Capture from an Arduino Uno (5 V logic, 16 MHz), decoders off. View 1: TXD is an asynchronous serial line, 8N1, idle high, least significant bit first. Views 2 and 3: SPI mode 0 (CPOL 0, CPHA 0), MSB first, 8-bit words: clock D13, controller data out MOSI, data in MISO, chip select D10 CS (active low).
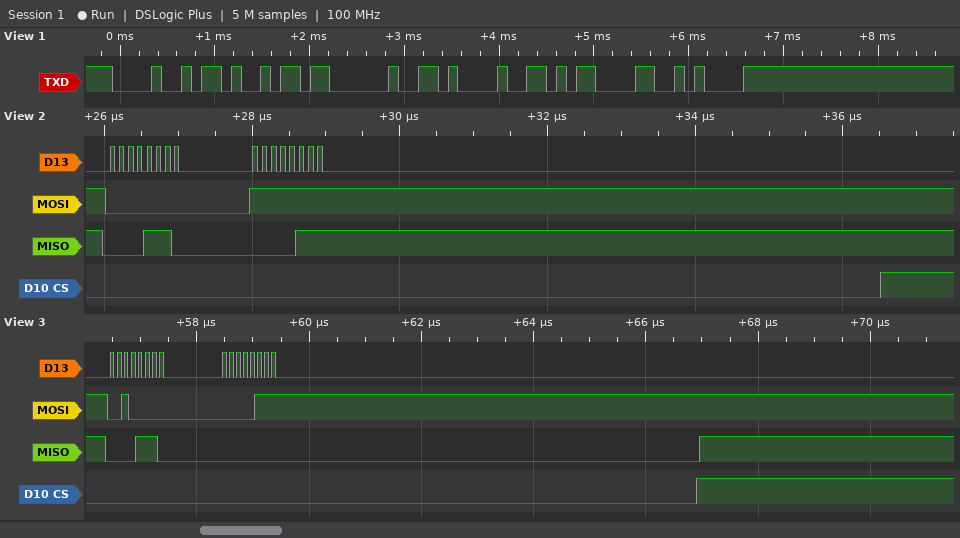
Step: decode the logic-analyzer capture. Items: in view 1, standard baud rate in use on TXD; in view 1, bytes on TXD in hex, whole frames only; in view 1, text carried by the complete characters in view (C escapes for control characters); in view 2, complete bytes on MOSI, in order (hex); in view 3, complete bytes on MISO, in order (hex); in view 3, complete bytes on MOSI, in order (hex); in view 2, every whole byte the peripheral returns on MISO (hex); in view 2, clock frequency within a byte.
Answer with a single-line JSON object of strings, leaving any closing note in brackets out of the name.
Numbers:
{"in view 1, standard baud rate in use on TXD": "9600 baud", "in view 1, bytes on TXD in hex, whole frames only": "48 69 20 21 0D 0A", "in view 1, text carried by the complete characters in view": "\"Hi !\\r\\n\"", "in view 2, complete bytes on MOSI, in order": "00 FF", "in view 3, complete bytes on MISO, in order": "0E 00", "in view 3, complete bytes on MOSI, in order": "20 07", "in view 2, every whole byte the peripheral returns on MISO": "0E 07", "in view 2, clock frequency within a byte": "8 MHz"}
